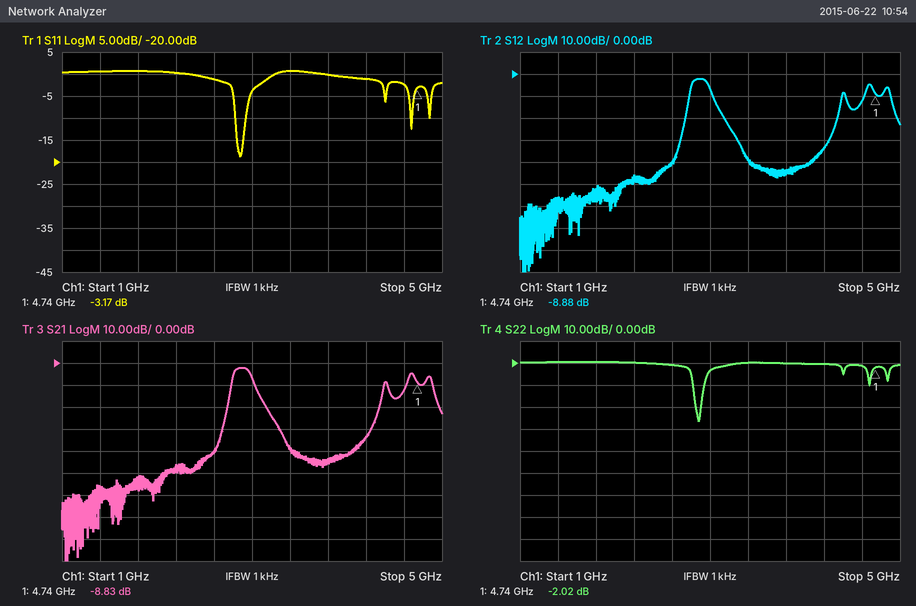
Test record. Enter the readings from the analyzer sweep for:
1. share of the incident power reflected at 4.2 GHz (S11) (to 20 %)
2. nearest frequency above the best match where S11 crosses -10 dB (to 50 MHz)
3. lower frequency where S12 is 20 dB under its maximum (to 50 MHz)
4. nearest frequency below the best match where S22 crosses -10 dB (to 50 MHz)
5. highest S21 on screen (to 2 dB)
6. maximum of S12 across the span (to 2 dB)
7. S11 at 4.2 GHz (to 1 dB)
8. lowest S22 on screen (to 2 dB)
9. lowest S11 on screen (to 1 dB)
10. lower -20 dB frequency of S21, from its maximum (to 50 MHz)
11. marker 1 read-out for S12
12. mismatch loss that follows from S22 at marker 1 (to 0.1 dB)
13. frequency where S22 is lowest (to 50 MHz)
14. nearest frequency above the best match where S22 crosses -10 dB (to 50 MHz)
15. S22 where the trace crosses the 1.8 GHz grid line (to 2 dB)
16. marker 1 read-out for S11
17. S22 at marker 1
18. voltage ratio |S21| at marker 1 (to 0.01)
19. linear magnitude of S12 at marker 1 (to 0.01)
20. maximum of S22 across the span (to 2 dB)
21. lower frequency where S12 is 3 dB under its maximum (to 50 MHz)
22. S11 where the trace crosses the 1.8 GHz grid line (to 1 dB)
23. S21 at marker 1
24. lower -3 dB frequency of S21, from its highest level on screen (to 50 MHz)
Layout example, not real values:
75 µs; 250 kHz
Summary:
80 %; 2.95 GHz; 2.75 GHz; 2.80 GHz; -2 dB; -2 dB; -1 dB; -26 dB; -19 dB; 2.75 GHz; -8.88 dB; 4.3 dB; 2.90 GHz; 2.95 GHz; 0 dB; -3.17 dB; -2.02 dB; 0.36; 0.36; 0 dB; 2.80 GHz; 1 dB; -8.83 dB; 2.80 GHz
